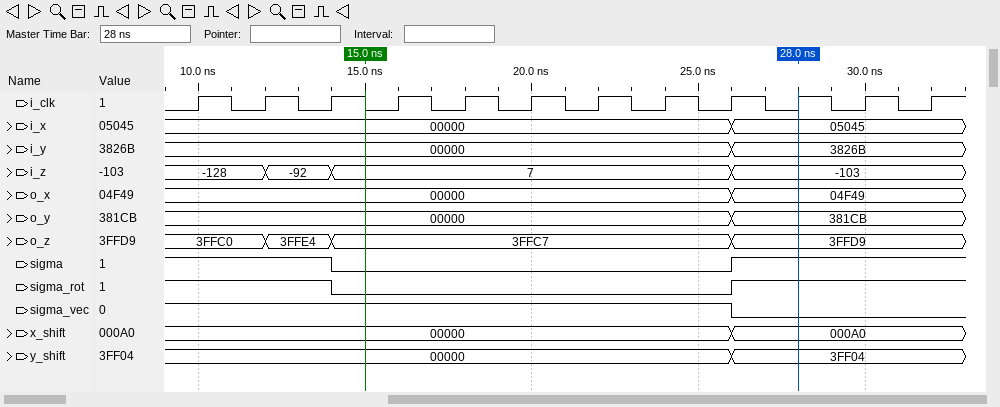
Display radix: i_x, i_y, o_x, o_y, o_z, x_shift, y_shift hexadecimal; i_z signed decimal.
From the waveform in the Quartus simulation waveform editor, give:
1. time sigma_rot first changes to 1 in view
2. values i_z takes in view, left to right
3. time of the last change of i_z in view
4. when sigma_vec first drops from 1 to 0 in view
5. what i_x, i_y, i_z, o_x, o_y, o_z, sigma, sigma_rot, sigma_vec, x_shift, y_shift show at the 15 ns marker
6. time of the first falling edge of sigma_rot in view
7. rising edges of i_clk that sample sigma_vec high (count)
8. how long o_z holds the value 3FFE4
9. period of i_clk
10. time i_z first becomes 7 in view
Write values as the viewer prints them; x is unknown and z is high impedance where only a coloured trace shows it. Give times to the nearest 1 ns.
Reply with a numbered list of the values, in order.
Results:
1. 26 ns
2. -128, -92, 7, -103
3. 26 ns
4. 26 ns
5. i_x=00000, i_y=00000, i_z=7, o_x=00000, o_y=00000, o_z=3FFC7, sigma=0, sigma_rot=0, sigma_vec=1, x_shift=00000, y_shift=00000
6. 14 ns
7. 9
8. 2 ns
9. 2 ns
10. 14 ns
